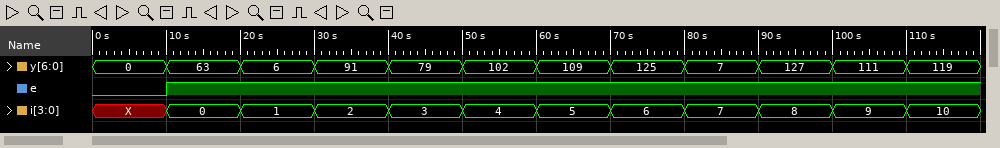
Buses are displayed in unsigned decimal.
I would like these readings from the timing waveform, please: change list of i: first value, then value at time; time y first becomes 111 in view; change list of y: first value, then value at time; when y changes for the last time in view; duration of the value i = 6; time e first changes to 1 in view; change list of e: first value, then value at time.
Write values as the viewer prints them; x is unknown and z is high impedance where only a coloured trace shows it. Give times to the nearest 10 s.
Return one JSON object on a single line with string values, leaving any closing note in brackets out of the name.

{"change list of i: first value, then value at time": "X, 0 at 10 s, 1 at 20 s, 2 at 30 s, 3 at 40 s, 4 at 50 s, 5 at 60 s, 6 at 70 s, 7 at 80 s, 8 at 90 s, 9 at 100 s, 10 at 110 s", "time y first becomes 111 in view": "100 s", "change list of y: first value, then value at time": "0, 63 at 10 s, 6 at 20 s, 91 at 30 s, 79 at 40 s, 102 at 50 s, 109 at 60 s, 125 at 70 s, 7 at 80 s, 127 at 90 s, 111 at 100 s, 119 at 110 s", "when y changes for the last time in view": "110 s", "duration of the value i = 6": "10 s", "time e first changes to 1 in view": "10 s", "change list of e: first value, then value at time": "0, 1 at 10 s"}
